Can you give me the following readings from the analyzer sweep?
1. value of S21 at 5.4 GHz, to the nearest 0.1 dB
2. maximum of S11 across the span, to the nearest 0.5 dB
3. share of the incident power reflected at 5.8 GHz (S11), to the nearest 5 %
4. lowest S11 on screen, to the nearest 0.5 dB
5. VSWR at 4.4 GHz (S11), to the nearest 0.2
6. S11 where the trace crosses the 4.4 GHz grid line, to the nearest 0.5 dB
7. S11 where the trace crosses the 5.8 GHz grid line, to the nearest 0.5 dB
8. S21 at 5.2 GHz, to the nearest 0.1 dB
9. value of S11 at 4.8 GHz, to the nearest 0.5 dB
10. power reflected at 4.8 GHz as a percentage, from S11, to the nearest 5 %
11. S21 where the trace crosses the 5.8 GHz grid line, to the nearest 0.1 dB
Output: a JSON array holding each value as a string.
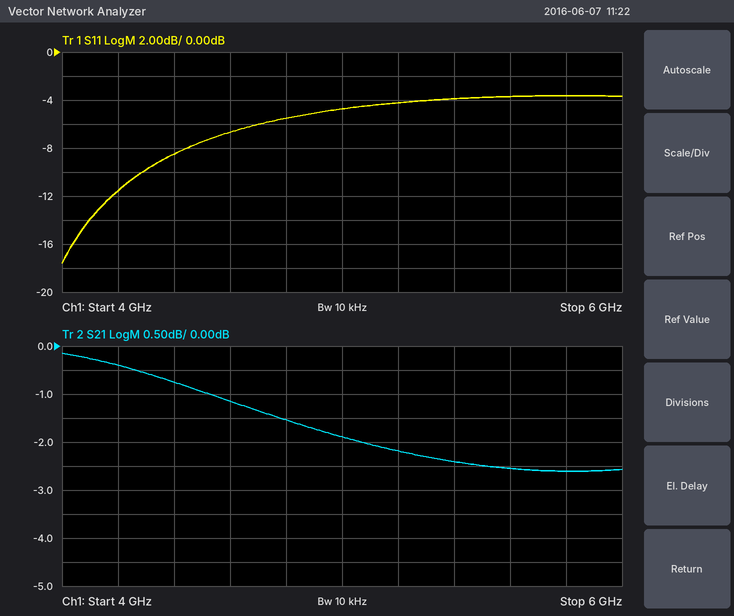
["-2.4 dB", "-3.5 dB", "45 %", "-17.5 dB", "2.2", "-8.5 dB", "-3.5 dB", "-2.2 dB", "-5.5 dB", "30 %", "-2.6 dB"]
